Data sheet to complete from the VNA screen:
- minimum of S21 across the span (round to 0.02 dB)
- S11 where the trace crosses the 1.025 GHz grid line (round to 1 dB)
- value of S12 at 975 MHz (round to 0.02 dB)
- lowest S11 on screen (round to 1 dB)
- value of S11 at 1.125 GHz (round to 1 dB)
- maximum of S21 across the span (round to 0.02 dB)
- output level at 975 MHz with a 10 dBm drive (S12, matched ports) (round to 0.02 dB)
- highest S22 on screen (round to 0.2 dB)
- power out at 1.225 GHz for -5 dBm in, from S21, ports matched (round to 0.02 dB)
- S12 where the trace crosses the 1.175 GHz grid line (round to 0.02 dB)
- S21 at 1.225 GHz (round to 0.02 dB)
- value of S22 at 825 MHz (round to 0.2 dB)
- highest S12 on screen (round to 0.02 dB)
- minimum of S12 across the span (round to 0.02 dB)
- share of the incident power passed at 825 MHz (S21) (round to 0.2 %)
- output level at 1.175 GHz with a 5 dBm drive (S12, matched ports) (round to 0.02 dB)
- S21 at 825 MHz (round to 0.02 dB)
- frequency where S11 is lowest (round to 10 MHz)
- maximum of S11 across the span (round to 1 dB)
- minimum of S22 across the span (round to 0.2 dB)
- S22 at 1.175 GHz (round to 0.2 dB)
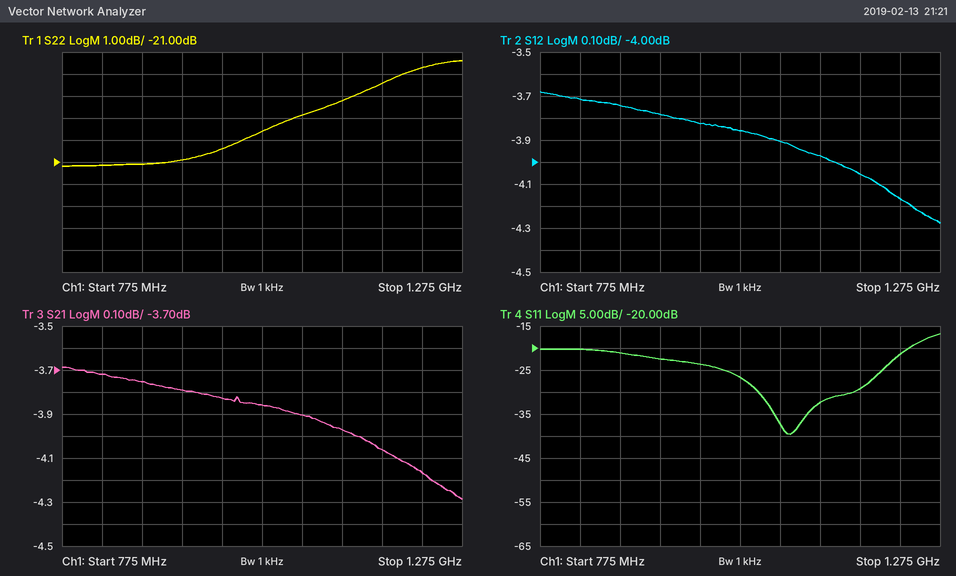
-4.28 dB
-27 dB
-3.82 dB
-40 dB
-32 dB
-3.68 dB
6.18 dBm
-16.4 dB
-9.16 dBm
-4.06 dB
-4.16 dB
-21.2 dB
-3.68 dB
-4.28 dB
42.4 %
0.94 dBm
-3.72 dB
1.09 GHz
-17 dB
-21.2 dB
-17.4 dB
